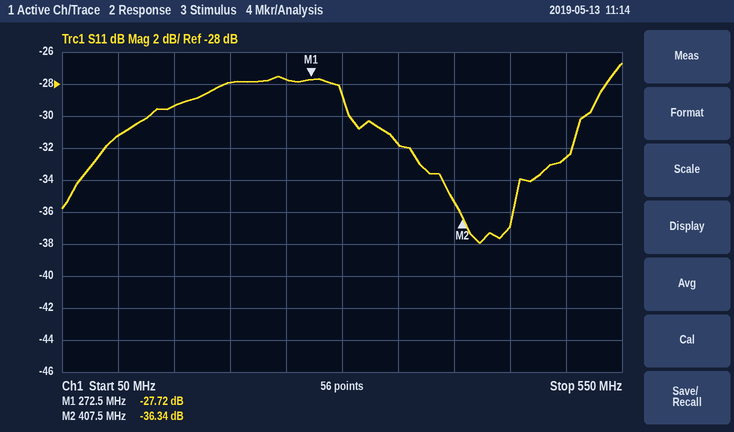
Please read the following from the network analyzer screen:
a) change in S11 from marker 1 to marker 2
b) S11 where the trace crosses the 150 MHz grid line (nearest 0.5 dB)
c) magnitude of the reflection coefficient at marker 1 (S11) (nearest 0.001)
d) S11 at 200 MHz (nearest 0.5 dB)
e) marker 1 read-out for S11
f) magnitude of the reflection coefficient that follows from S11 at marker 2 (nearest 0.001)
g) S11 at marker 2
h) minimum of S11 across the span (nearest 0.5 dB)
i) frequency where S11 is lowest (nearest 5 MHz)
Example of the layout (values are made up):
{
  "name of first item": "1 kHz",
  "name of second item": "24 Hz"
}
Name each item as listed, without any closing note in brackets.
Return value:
{
  "change in S11 from marker 1 to marker 2": "-8.62 dB",
  "S11 where the trace crosses the 150 MHz grid line": "-29.5 dB",
  "magnitude of the reflection coefficient at marker 1 (S11)": "0.041",
  "S11 at 200 MHz": "-28.0 dB",
  "marker 1 read-out for S11": "-27.72 dB",
  "magnitude of the reflection coefficient that follows from S11 at marker 2": "0.015",
  "S11 at marker 2": "-36.34 dB",
  "minimum of S11 across the span": "-38.0 dB",
  "frequency where S11 is lowest": "425 MHz"
}
